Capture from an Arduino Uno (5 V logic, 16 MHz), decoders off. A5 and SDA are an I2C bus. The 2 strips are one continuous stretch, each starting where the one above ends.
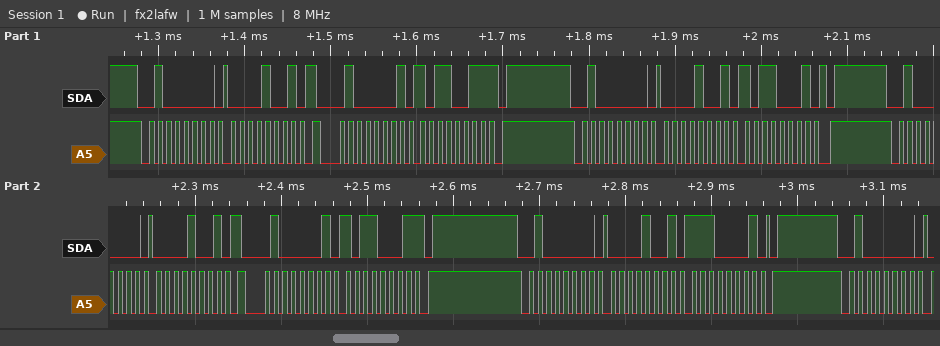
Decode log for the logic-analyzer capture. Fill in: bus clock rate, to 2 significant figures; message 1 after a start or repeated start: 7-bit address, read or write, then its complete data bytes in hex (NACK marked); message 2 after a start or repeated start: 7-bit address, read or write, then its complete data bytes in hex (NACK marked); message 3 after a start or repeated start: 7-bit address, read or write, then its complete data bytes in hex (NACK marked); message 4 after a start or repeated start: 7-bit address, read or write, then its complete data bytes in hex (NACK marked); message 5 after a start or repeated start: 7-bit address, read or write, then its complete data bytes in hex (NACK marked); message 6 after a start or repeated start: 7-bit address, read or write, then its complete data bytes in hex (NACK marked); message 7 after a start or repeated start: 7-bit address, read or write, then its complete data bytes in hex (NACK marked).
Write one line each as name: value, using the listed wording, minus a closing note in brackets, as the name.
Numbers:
bus clock rate, to 2 significant figures: 100 kHz
message 1 after a start or repeated start: 7-bit address, read or write, then its complete data bytes in hex: 0x20 write: 09
message 2 after a start or repeated start: 7-bit address, read or write, then its complete data bytes in hex: 0x20 read: B3 NACK
message 3 after a start or repeated start: 7-bit address, read or write, then its complete data bytes in hex: 0x20 write: 09 B1
message 4 after a start or repeated start: 7-bit address, read or write, then its complete data bytes in hex: 0x20 write: 09
message 5 after a start or repeated start: 7-bit address, read or write, then its complete data bytes in hex: 0x20 read: B1 NACK
message 6 after a start or repeated start: 7-bit address, read or write, then its complete data bytes in hex: 0x20 write: 09 E1
message 7 after a start or repeated start: 7-bit address, read or write, then its complete data bytes in hex: 0x20 write
